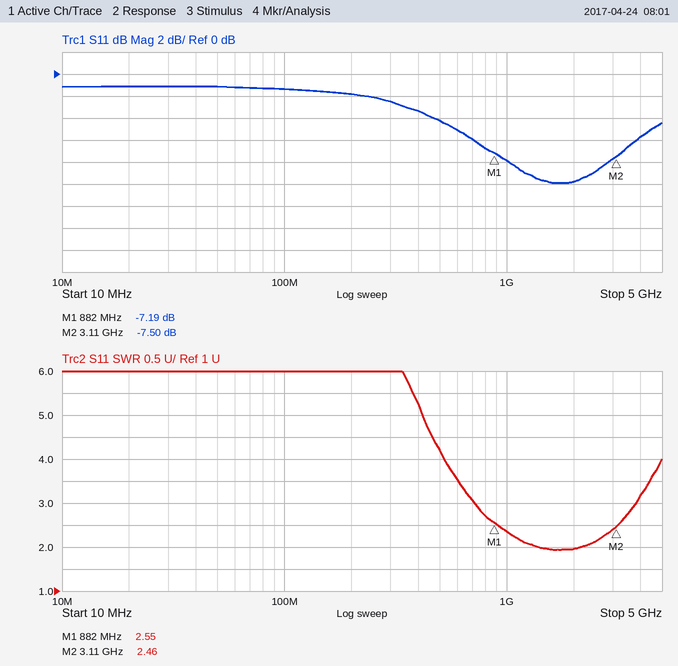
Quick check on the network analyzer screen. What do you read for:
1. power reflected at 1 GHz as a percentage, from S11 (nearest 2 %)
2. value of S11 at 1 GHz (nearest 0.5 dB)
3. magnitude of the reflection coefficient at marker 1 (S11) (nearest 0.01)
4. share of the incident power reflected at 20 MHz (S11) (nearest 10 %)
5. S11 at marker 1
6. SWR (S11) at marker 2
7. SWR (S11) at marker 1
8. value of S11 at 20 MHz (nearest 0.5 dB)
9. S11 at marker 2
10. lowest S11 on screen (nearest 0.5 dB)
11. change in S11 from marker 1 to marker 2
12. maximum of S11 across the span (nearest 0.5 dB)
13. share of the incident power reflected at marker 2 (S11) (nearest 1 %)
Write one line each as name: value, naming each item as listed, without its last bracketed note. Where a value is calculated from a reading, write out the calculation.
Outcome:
power reflected at 1 GHz as a percentage, from S11: 10^(-8/10) ≈ 16 %
value of S11 at 1 GHz: -8.0 dB
magnitude of the reflection coefficient at marker 1 (S11): 10^(-7.19/20) ≈ 0.44
share of the incident power reflected at 20 MHz (S11): 10^(-1/10) ≈ 79.4 %, so 80 % to the nearest 10 %
S11 at marker 1: -7.19 dB
SWR (S11) at marker 2: 2.46
SWR (S11) at marker 1: 2.55
value of S11 at 20 MHz: -1.0 dB
S11 at marker 2: -7.50 dB
lowest S11 on screen: -10.0 dB
change in S11 from marker 1 to marker 2: -7.5 − (-7.19) = -0.31 dB
maximum of S11 across the span: -1.0 dB
share of the incident power reflected at marker 2 (S11): 10^(-7.5/10) ≈ 18 %
